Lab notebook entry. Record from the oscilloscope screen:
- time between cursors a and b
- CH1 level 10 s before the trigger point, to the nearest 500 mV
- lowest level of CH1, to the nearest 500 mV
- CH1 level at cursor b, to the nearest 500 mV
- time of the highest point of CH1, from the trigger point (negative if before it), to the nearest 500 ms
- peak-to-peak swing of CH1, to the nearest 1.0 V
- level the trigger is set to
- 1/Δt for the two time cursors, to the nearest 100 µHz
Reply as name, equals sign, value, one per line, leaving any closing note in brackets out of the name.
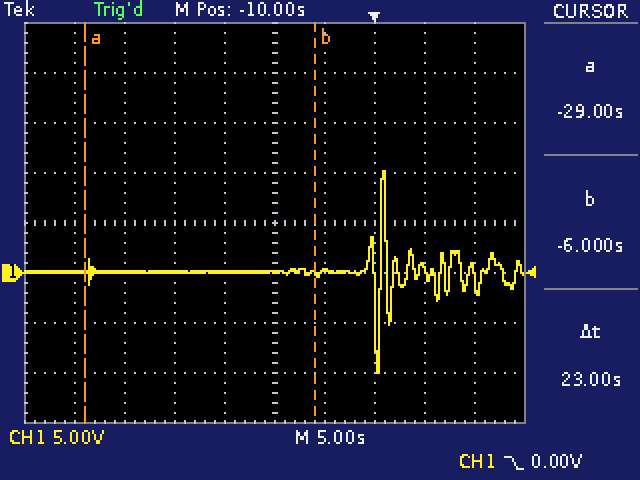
time between cursors a and b = 23 s
CH1 level 10 s before the trigger point, to the nearest 500 mV = 0.0 V
lowest level of CH1, to the nearest 500 mV = -10.0 V
CH1 level at cursor b, to the nearest 500 mV = 0.0 V
time of the highest point of CH1, from the trigger point (negative if before it), to the nearest 500 ms = +1.0 s
peak-to-peak swing of CH1, to the nearest 1.0 V = 20.0 V
level the trigger is set to = 0.00 V
1/Δt for the two time cursors, to the nearest 100 µHz = 43.5 mHz
